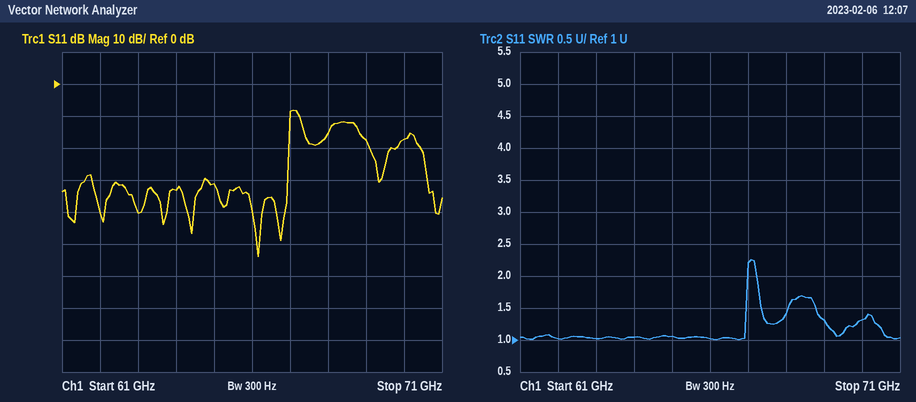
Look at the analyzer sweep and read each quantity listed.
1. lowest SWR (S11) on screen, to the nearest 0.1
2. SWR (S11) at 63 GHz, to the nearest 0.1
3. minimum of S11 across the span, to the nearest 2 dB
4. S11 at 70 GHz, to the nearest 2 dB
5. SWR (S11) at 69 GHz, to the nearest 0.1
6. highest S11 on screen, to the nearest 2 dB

1.0
1.0
-54 dB
-18 dB
1.3
-8 dB
